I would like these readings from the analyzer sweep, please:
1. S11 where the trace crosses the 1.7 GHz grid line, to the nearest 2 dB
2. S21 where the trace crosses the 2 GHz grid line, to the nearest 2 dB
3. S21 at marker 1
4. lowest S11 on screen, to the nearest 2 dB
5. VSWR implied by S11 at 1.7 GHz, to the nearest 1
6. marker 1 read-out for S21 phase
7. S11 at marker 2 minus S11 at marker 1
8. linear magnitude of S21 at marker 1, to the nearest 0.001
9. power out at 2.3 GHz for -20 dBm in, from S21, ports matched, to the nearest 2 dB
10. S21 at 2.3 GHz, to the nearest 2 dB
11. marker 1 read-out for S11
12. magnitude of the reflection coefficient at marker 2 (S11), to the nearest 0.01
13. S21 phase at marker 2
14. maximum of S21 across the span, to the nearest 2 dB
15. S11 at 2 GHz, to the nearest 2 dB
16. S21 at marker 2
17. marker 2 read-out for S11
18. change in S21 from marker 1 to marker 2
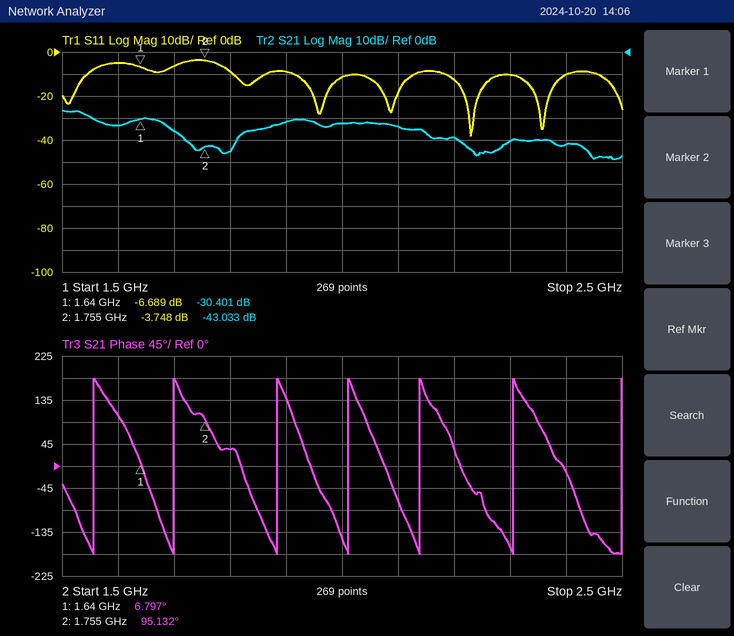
-6 dB
-32 dB
-30.401 dB
-38 dB
3
6.797°
2.941 dB
0.030
-60 dBm
-40 dB
-6.689 dB
0.65
95.132°
-26 dB
-12 dB
-43.033 dB
-3.748 dB
-12.632 dB
